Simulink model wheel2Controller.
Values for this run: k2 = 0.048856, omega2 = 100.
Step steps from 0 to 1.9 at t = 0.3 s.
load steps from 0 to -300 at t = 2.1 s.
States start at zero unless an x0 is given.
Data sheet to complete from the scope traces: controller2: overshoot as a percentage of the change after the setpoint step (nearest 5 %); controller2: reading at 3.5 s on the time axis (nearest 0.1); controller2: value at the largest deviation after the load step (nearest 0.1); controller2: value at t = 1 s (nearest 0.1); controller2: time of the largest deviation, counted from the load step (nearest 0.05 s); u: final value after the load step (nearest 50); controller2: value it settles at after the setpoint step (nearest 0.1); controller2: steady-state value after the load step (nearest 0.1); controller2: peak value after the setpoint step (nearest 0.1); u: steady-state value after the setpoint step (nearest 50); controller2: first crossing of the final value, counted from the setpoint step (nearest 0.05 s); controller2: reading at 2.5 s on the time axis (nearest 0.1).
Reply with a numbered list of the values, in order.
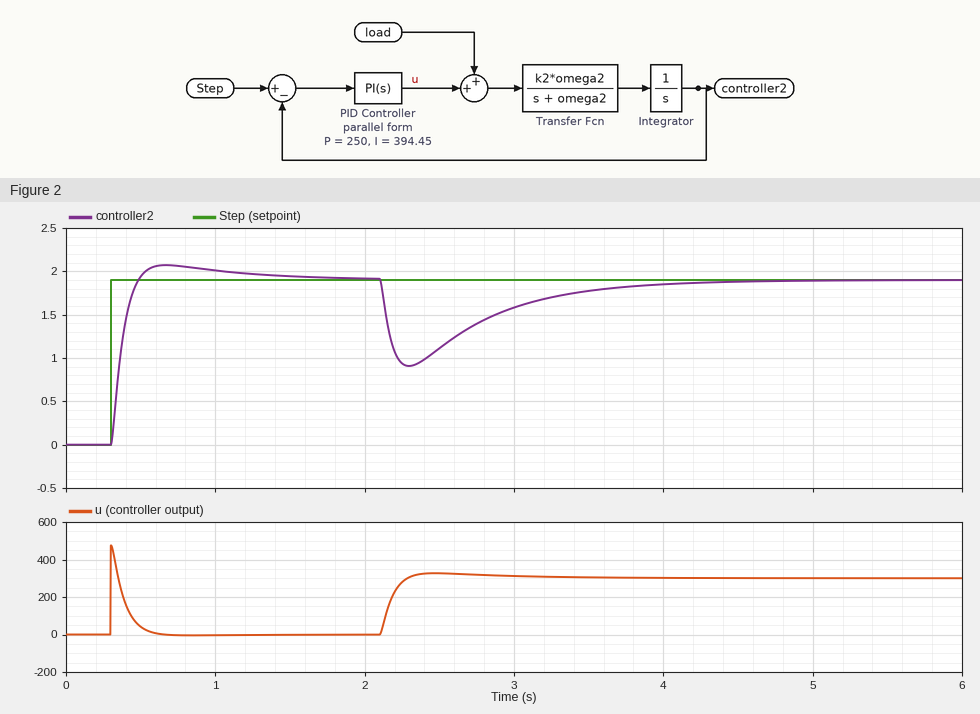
1. 10 %
2. 1.8
3. 0.9
4. 2.0
5. 0.20 s
6. 300
7. 1.9
8. 1.9
9. 2.1
10. 0
11. 0.20 s
12. 1.1
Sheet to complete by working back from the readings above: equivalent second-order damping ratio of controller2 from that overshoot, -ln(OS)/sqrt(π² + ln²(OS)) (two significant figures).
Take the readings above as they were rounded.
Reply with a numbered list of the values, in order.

1. 0.59
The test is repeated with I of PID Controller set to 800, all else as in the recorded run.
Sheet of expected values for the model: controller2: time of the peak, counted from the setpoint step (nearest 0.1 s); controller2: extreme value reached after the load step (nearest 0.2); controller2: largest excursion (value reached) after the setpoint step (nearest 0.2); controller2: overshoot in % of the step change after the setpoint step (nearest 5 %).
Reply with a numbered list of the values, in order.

1. 0.3 s
2. 1.0
3. 2.2
4. 15 %
